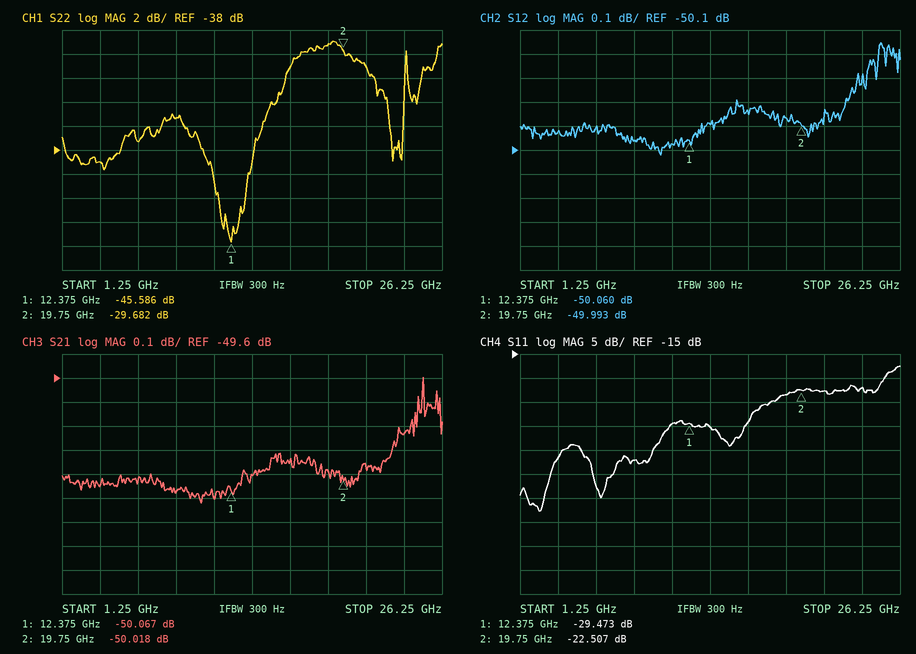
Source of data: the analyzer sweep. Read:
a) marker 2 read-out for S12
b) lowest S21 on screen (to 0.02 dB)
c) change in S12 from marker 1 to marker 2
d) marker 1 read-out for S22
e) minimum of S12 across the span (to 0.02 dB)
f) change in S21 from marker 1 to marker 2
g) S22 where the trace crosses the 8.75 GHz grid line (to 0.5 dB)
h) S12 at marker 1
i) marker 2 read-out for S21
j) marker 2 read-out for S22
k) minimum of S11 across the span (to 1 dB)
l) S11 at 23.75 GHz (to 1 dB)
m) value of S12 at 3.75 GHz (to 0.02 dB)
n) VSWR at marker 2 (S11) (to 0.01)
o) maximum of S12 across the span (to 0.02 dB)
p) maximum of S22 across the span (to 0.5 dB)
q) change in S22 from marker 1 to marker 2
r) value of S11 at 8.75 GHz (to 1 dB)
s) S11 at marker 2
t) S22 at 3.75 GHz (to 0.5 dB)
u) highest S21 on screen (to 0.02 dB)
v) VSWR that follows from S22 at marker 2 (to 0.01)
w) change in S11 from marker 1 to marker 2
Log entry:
-49.993 dB
-50.12 dB
0.067 dB
-45.586 dB
-50.12 dB
0.049 dB
-35.5 dB
-50.060 dB
-50.018 dB
-29.682 dB
-48 dB
-22 dB
-50.02 dB
1.16
-49.66 dB
-29.0 dB
15.904 dB
-37 dB
-22.507 dB
-39.0 dB
-49.60 dB
1.07
6.966 dB
